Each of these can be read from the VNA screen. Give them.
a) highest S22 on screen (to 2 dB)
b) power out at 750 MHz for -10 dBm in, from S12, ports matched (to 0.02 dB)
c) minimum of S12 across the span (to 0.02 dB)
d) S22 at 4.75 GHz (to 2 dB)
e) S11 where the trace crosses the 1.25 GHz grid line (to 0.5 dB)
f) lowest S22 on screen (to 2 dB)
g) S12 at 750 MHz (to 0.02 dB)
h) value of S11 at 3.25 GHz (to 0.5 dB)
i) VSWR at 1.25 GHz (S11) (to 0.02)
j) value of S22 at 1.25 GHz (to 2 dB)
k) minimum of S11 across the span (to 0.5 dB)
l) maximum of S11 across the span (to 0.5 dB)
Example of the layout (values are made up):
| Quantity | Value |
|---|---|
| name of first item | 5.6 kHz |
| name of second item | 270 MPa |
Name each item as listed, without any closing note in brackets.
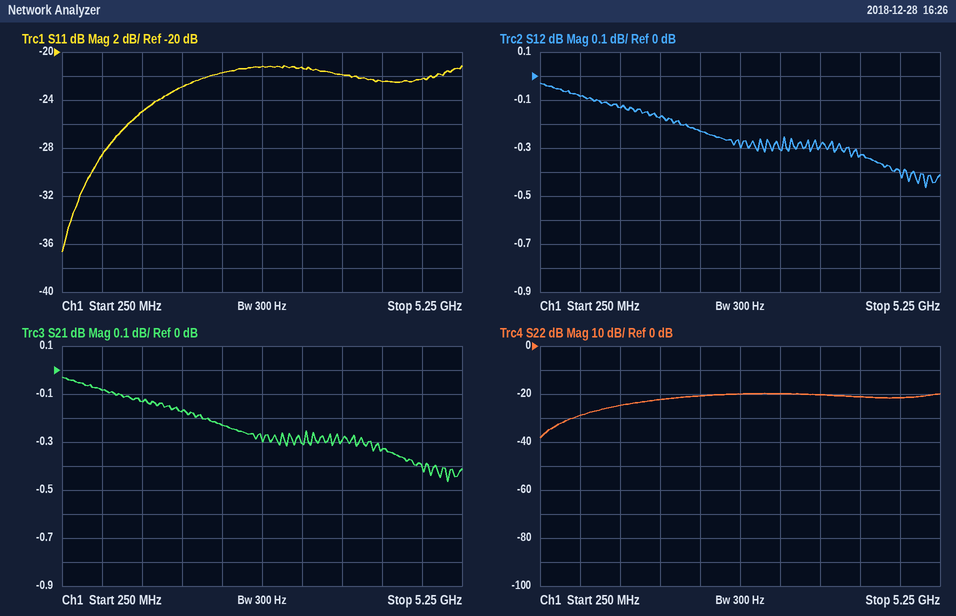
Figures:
| Quantity | Value |
|---|---|
| highest S22 on screen | -20 dB |
| power out at 750 MHz for -10 dBm in, from S12, ports matched | -10.08 dBm |
| minimum of S12 across the span | -0.46 dB |
| S22 at 4.75 GHz | -22 dB |
| S11 where the trace crosses the 1.25 GHz grid line | -25.0 dB |
| lowest S22 on screen | -38 dB |
| S12 at 750 MHz | -0.08 dB |
| value of S11 at 3.25 GHz | -21.5 dB |
| VSWR at 1.25 GHz (S11) | 1.12 |
| value of S22 at 1.25 GHz | -24 dB |
| minimum of S11 across the span | -36.5 dB |
| maximum of S11 across the span | -21.0 dB |
